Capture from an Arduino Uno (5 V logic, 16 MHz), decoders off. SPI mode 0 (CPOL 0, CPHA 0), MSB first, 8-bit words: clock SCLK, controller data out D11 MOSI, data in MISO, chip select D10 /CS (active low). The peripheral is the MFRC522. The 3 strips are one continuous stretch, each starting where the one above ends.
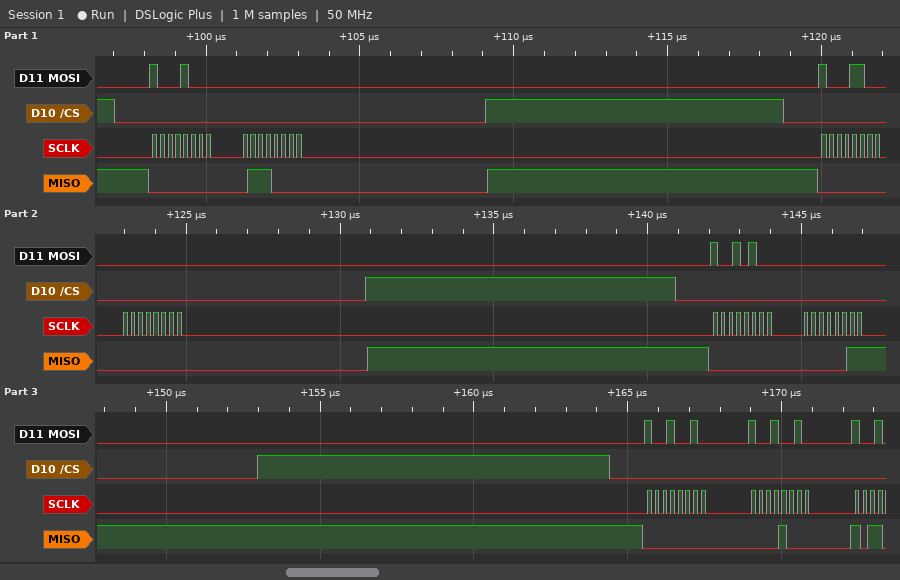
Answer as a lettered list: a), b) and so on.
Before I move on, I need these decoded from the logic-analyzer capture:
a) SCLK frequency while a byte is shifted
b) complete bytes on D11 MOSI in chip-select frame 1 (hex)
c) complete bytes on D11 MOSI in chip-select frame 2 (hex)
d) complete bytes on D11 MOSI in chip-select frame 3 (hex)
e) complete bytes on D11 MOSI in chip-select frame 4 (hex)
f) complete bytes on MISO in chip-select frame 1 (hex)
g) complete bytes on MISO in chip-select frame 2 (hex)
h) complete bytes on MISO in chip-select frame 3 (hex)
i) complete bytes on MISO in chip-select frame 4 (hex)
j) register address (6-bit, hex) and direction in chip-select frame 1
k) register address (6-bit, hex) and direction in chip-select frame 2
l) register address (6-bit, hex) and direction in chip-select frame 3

a) 4 MHz
b) 0x88 0x00
c) 0x8C 0x00
d) 0x94 0x00
e) 0x92 0x92
f) 0x00 0x70
g) 0x00 0x00
h) 0x00 0x03
i) 0x00 0x08
j) 0x04 read
k) 0x06 read
l) 0x0A read
